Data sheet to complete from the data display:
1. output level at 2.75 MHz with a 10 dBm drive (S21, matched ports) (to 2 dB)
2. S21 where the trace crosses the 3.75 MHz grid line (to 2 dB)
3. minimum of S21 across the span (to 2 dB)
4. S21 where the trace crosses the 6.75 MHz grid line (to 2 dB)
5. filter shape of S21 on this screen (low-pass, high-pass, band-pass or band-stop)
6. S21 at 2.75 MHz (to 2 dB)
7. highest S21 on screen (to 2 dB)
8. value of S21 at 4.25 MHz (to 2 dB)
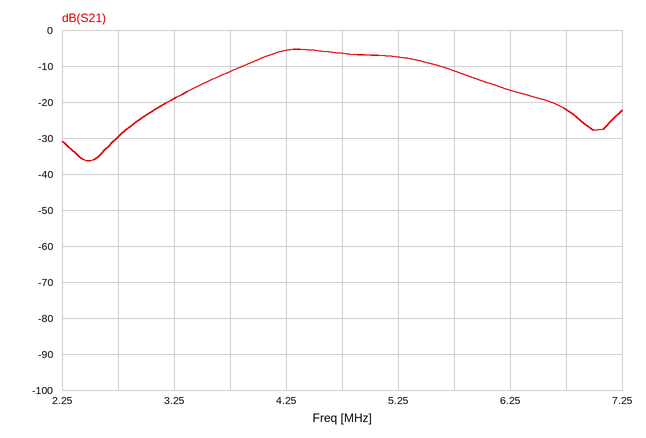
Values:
-20 dBm
-12 dB
-36 dB
-22 dB
band-pass
-30 dB
-6 dB
-6 dB
